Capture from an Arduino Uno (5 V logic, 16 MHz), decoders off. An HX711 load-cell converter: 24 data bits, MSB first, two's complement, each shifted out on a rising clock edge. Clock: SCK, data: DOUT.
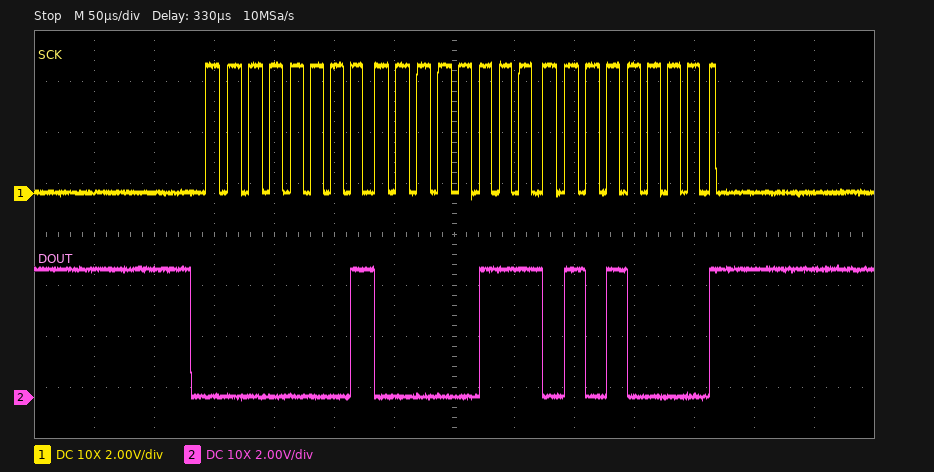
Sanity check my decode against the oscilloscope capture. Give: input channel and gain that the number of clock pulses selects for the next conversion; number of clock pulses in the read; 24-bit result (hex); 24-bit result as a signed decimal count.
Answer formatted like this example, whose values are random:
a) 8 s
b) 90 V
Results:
a) channel A, gain 128
b) 25
c) 0x010750
d) 67408
